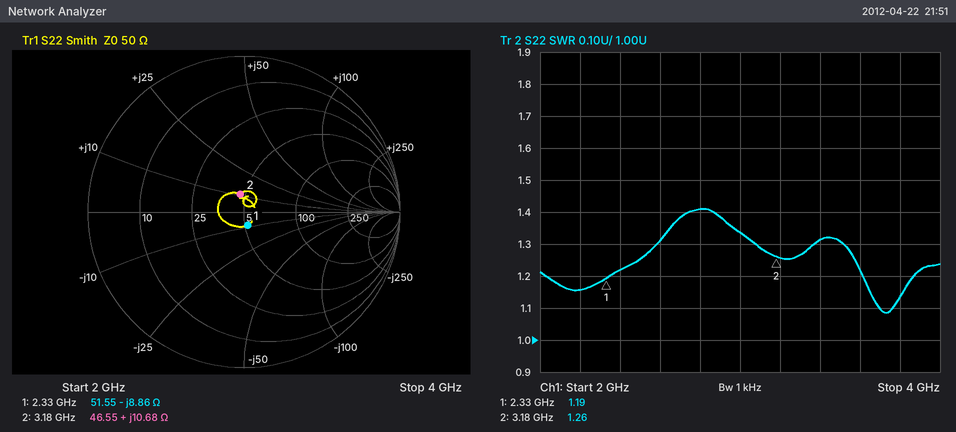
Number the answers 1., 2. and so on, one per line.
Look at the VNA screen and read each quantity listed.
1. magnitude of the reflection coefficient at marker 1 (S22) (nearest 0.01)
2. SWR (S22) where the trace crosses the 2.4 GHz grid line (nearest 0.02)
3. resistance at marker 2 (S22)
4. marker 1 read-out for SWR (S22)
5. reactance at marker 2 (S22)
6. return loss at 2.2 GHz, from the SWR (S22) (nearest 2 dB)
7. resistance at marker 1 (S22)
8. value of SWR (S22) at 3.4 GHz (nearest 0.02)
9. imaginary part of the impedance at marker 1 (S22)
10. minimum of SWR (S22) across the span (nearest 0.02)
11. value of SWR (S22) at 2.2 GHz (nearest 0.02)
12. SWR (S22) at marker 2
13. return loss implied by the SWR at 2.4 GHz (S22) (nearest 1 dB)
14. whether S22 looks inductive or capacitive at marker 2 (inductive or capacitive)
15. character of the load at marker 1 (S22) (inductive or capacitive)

1. 0.09
2. 1.22
3. 46.55 Ω
4. 1.19
5. +10.68 Ω
6. 22 dB
7. 51.55 Ω
8. 1.32
9. -8.86 Ω
10. 1.08
11. 1.16
12. 1.26
13. 20 dB
14. inductive
15. capacitive
